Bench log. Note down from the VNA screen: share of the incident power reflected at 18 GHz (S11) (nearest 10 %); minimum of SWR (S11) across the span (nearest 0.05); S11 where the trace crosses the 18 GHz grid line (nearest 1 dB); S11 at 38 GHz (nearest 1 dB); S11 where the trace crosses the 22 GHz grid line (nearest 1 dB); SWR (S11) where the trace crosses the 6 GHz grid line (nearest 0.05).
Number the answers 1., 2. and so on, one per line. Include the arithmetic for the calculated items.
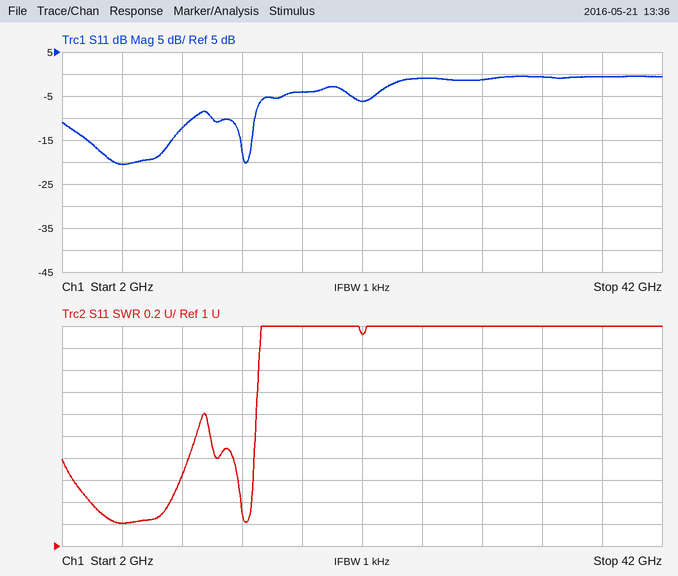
1. 10^(-4/10) ≈ 40 %
2. 1.20
3. -4 dB
4. -1 dB
5. -6 dB
6. 1.20
